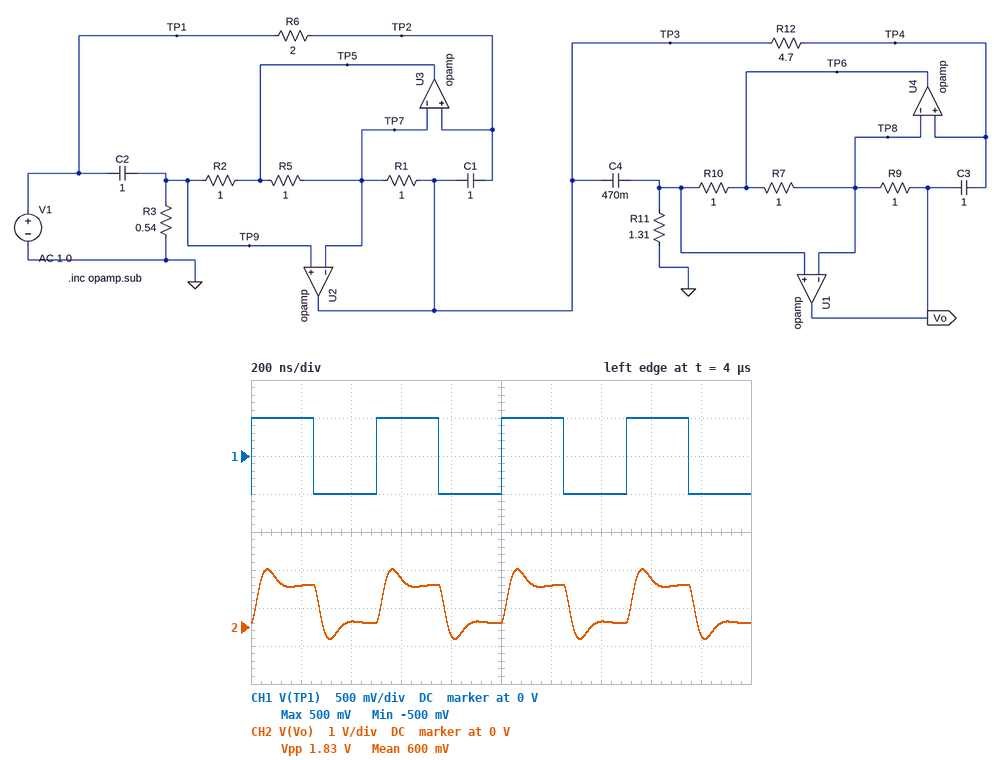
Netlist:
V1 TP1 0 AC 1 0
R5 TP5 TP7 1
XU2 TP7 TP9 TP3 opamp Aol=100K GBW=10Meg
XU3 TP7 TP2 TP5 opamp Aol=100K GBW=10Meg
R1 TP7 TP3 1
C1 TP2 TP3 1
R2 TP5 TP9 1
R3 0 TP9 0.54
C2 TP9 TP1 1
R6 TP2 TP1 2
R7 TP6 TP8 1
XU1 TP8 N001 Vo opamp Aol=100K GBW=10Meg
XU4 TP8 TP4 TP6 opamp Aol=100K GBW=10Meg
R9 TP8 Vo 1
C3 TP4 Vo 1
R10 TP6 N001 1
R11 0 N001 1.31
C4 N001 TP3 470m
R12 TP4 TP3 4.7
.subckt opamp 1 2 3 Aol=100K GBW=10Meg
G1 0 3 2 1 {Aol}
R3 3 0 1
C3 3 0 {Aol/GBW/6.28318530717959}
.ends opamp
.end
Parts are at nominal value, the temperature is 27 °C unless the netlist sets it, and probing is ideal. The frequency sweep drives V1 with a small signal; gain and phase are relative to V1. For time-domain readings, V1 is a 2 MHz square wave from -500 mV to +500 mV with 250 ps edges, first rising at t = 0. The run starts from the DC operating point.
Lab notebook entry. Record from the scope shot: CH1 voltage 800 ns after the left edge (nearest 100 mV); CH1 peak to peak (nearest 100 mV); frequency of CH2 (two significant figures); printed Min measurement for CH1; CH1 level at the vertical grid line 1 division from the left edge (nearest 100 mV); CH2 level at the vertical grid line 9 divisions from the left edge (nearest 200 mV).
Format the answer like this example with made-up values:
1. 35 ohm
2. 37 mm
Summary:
1. -500 mV
2. 1.0 V
3. 2.0 MHz
4. -500 mV
5. 500 mV
6. -200 mV
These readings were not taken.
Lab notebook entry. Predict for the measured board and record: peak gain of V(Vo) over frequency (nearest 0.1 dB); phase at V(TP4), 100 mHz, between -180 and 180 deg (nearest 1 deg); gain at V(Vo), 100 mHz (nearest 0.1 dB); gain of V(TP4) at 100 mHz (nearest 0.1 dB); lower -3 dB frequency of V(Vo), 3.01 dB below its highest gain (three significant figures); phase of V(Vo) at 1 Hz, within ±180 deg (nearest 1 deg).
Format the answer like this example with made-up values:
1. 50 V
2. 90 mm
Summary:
1. 0 dB
2. 8 deg
3. -14.1 dB
4. -28.0 dB
5. 322 mHz
6. 31 deg
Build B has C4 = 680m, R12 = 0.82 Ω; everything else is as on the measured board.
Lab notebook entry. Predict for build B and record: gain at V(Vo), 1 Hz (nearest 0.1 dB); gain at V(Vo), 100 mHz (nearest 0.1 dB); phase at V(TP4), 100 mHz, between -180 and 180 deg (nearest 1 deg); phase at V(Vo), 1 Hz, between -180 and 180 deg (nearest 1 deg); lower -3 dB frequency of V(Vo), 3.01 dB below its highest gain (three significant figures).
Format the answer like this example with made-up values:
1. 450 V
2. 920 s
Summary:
1. 0 dB
2. -37.5 dB
3. 68 deg
4. 27 deg
5. 211 mHz
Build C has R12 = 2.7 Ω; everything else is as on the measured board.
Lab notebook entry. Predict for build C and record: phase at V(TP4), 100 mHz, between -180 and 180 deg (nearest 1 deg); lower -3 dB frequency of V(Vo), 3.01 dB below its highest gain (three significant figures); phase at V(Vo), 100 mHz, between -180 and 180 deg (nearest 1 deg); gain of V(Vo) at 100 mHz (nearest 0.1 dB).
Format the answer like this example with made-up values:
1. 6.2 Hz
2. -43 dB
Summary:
1. 26 deg
2. 305 mHz
3. -154 deg
4. -17.5 dB
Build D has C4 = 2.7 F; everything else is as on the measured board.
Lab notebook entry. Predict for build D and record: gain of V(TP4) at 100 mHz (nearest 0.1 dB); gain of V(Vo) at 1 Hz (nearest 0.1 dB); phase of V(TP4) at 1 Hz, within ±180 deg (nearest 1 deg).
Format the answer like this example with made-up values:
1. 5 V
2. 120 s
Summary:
1. -4.3 dB
2. -0.2 dB
3. 19 deg
